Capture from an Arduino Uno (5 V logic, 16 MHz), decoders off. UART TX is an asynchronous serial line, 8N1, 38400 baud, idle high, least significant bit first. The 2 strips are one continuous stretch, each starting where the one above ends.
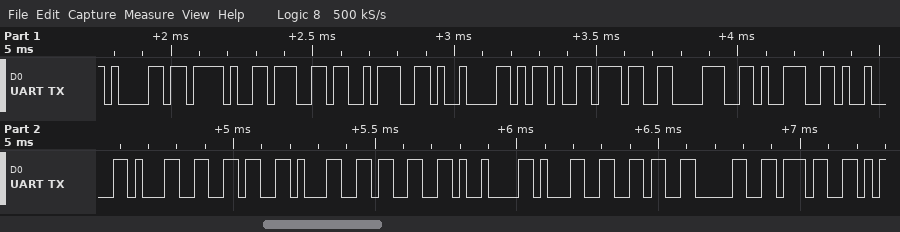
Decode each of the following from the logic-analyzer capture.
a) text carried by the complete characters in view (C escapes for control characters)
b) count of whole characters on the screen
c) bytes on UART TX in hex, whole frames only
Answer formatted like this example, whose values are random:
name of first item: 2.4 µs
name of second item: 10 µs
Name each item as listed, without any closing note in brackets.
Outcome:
text carried by the complete characters in view: "a/g:\t-789\t1613\t1607"
count of whole characters on the screen: 19
bytes on UART TX in hex, whole frames only: 61 2F 67 3A 09 2D 37 38 39 09 31 36 31 33 09 31 36 30 37
